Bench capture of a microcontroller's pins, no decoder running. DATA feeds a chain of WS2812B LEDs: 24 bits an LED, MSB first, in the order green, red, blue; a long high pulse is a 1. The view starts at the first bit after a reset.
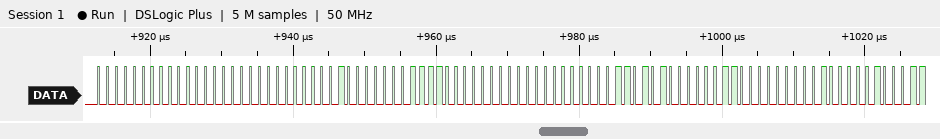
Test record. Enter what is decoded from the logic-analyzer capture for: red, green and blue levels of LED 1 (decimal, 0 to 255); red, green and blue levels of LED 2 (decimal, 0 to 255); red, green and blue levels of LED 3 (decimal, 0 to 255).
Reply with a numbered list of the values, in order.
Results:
1. 0, 0, 0
2. 30, 16, 0
3. 53, 0, 3
